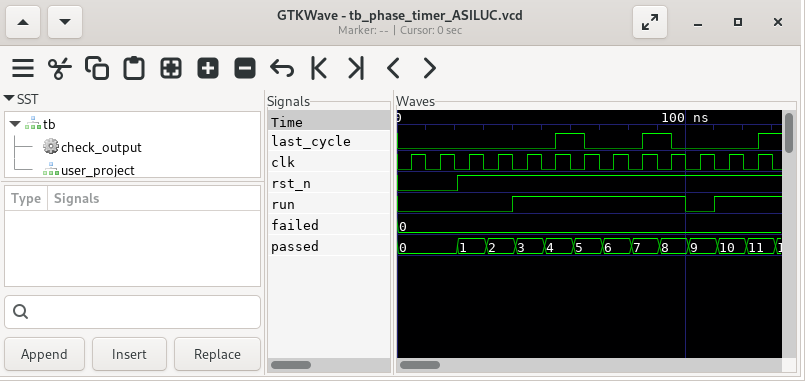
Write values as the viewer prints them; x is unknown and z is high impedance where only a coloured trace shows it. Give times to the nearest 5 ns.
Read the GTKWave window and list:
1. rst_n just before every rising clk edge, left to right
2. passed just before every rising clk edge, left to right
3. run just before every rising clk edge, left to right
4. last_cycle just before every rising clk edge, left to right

0 0 1 1 1 1 1 1 1 1 1 1 1
0, 0, 1, 2, 3, 4, 5, 6, 7, 8, 9, 10, 11
0 0 0 0 1 1 1 1 1 1 0 1 1
0 0 0 0 0 0 1 0 0 1 0 0 0
